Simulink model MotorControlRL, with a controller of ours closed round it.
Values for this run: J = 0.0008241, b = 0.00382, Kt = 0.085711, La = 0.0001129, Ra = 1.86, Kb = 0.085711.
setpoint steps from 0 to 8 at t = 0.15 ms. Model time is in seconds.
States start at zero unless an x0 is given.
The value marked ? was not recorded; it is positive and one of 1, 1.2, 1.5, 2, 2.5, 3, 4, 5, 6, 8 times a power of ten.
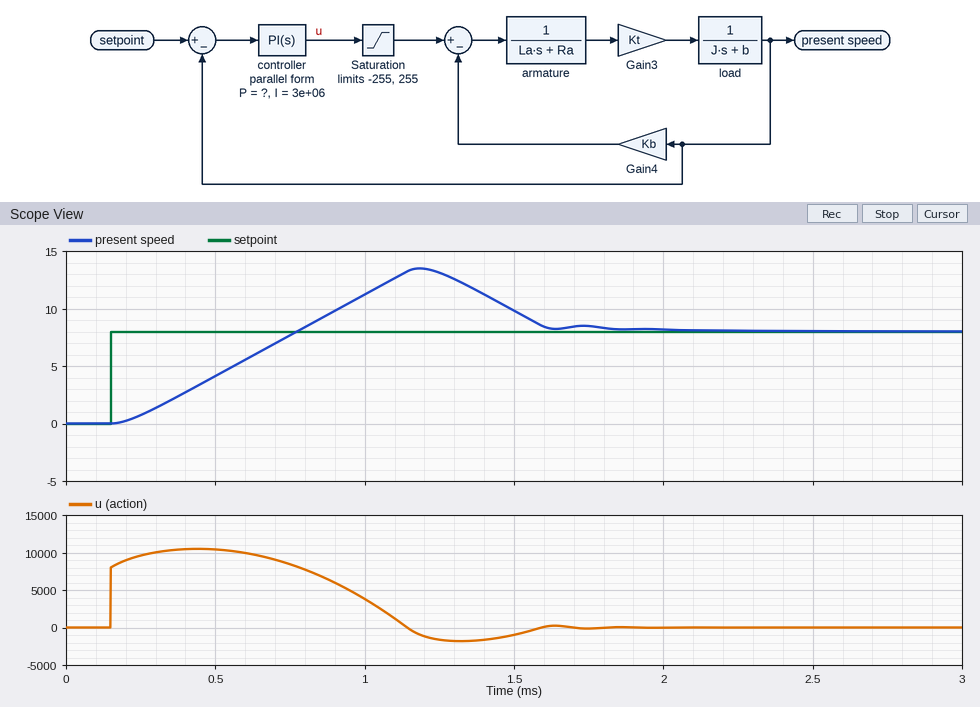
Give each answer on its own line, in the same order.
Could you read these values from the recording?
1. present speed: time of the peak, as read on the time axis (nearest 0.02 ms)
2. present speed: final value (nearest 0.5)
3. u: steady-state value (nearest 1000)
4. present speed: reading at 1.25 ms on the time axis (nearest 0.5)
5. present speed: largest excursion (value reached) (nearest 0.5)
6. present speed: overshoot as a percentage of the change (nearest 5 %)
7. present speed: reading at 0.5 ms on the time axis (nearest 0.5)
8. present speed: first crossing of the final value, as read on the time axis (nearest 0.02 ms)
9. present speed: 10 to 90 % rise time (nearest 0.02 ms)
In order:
1.18 ms
8.0
0
13.0
13.5
70 %
4.0
0.78 ms
0.46 ms
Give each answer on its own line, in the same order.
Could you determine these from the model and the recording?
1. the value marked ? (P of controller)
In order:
1000
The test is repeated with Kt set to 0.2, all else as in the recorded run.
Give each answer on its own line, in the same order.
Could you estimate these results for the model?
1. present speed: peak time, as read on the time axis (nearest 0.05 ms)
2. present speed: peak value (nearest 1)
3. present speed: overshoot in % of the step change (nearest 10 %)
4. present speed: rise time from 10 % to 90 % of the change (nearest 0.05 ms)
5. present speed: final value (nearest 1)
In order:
0.60 ms
12
50 %
0.20 ms
8
